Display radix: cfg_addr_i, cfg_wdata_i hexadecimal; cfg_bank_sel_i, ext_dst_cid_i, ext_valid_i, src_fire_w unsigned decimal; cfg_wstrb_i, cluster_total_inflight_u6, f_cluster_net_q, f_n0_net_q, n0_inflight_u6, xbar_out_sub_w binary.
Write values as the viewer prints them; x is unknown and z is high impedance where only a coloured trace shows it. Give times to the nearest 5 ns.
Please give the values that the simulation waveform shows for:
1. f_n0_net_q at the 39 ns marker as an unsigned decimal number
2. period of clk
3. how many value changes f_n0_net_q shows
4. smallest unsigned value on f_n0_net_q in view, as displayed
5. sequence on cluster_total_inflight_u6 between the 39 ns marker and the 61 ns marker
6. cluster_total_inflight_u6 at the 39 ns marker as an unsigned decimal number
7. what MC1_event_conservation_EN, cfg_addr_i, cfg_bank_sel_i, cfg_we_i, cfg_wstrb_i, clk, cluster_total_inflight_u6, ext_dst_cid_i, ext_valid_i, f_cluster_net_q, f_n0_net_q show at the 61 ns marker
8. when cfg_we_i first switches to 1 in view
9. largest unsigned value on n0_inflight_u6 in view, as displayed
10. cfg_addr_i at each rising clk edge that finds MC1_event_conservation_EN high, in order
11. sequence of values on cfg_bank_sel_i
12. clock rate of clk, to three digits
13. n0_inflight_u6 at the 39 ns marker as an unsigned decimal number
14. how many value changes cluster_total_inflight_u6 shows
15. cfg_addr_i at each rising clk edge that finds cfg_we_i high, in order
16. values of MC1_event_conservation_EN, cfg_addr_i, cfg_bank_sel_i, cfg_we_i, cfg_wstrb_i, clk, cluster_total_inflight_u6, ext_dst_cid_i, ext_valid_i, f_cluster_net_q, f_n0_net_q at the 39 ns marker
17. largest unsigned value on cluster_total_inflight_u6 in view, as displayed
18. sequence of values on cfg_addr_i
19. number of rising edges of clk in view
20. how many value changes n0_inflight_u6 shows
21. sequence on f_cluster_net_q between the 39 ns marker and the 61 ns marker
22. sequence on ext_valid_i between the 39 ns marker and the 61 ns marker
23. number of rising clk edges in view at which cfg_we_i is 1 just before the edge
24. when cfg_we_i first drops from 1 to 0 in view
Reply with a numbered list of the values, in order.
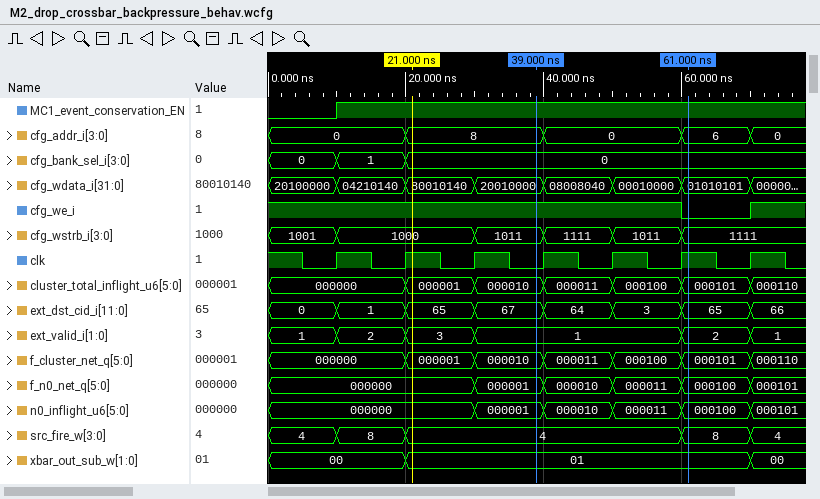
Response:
1. 1
2. 10 ns
3. 5
4. 000000
5. 000010, 000011, 000100, 000101
6. 2
7. MC1_event_conservation_EN=1, cfg_addr_i=6, cfg_bank_sel_i=0, cfg_we_i=0, cfg_wstrb_i=1111, clk=1, cluster_total_inflight_u6=000101, ext_dst_cid_i=65, ext_valid_i=2, f_cluster_net_q=000101, f_n0_net_q=000100
8. 70 ns
9. 000101
10. 0, 8, 8, 0, 0, 6
11. 0, 1, 0
12. 100 MHz
13. 1
14. 6
15. 0, 0, 8, 8, 0, 0
16. MC1_event_conservation_EN=1, cfg_addr_i=8, cfg_bank_sel_i=0, cfg_we_i=1, cfg_wstrb_i=1011, clk=0, cluster_total_inflight_u6=000010, ext_dst_cid_i=67, ext_valid_i=1, f_cluster_net_q=000010, f_n0_net_q=000001
17. 000110
18. 0, 8, 0, 6, 0
19. 7
20. 5
21. 000010, 000011, 000100, 000101
22. 1, 2
23. 6
24. 60 ns
